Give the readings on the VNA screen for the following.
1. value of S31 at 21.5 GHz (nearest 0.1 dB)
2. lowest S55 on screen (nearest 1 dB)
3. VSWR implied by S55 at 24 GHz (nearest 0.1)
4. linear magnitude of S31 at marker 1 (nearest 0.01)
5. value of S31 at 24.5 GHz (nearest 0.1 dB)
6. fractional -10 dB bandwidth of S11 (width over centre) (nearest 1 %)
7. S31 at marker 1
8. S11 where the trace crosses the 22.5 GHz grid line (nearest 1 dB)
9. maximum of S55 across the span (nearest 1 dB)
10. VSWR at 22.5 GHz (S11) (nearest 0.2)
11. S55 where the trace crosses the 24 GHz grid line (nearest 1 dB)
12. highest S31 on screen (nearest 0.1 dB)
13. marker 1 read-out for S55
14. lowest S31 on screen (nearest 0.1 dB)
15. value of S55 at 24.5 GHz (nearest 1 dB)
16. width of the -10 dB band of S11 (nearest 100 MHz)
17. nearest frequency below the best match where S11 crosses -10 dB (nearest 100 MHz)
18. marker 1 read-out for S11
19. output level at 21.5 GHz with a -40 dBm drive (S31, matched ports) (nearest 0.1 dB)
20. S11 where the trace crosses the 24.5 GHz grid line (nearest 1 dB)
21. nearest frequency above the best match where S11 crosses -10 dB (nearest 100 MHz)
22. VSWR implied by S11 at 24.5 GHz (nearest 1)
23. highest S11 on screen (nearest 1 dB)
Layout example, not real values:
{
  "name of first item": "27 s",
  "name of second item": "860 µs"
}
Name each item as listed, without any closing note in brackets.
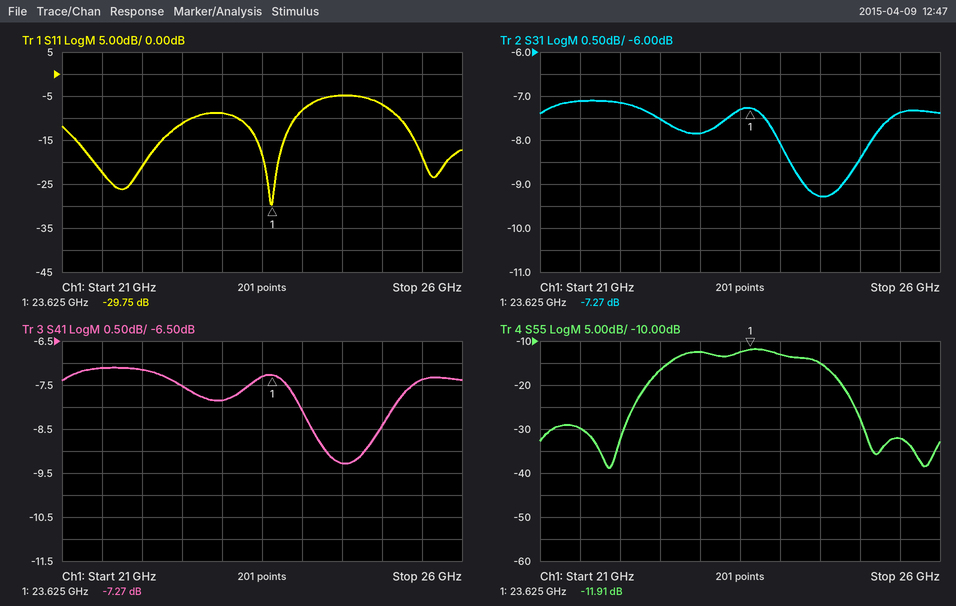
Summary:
{
  "value of S31 at 21.5 GHz": "-7.1 dB",
  "lowest S55 on screen": "-39 dB",
  "VSWR implied by S55 at 24 GHz": "1.6",
  "linear magnitude of S31 at marker 1": "0.43",
  "value of S31 at 24.5 GHz": "-9.3 dB",
  "fractional -10 dB bandwidth of S11 (width over centre)": "3 %",
  "S31 at marker 1": "-7.27 dB",
  "S11 where the trace crosses the 22.5 GHz grid line": "-11 dB",
  "maximum of S55 across the span": "-12 dB",
  "VSWR at 22.5 GHz (S11)": "1.8",
  "S55 where the trace crosses the 24 GHz grid line": "-13 dB",
  "highest S31 on screen": "-7.1 dB",
  "marker 1 read-out for S55": "-11.91 dB",
  "lowest S31 on screen": "-9.3 dB",
  "value of S55 at 24.5 GHz": "-15 dB",
  "width of the -10 dB band of S11": "700 MHz",
  "nearest frequency below the best match where S11 crosses -10 dB": "23.2 GHz",
  "marker 1 read-out for S11": "-29.75 dB",
  "output level at 21.5 GHz with a -40 dBm drive (S31, matched ports)": "-47.1 dBm",
  "S11 where the trace crosses the 24.5 GHz grid line": "-5 dB",
  "nearest frequency above the best match where S11 crosses -10 dB": "23.9 GHz",
  "VSWR implied by S11 at 24.5 GHz": "4",
  "highest S11 on screen": "-5 dB"
}
